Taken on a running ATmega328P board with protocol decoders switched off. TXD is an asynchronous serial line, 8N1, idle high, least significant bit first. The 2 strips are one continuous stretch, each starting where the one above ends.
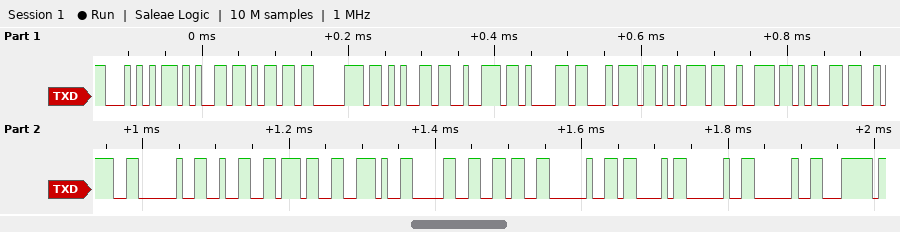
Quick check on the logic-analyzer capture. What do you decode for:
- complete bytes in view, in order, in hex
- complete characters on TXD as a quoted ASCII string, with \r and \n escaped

54 65 6D 70 65 72 61 74 75 72 65 3A 20 32 37 2E 30 36 20 43 20 20 7C
"Temperature: 27.06 C  |"
